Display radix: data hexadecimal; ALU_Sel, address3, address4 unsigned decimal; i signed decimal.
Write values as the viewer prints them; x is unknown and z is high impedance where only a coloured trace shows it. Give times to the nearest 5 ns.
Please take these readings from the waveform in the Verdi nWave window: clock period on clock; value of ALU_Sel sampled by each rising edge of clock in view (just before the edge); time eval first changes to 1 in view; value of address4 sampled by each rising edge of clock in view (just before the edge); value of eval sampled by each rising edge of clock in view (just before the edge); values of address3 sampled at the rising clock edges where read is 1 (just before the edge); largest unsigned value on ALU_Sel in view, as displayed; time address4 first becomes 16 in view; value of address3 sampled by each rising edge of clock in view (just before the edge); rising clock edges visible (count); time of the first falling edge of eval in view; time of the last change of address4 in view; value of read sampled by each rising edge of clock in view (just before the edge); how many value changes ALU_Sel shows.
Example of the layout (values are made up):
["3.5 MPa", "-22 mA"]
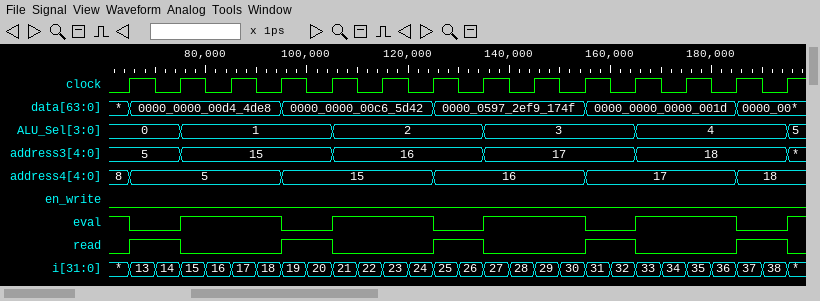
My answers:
["10 ns", "0, 0, 1, 1, 1, 2, 2, 2, 3, 3, 3, 4, 4, 4", "75 ns", "8, 5, 5, 5, 15, 15, 15, 16, 16, 16, 17, 17, 17, 18", "1 0 1 1 0 1 1 0 1 1 0 1 1 0", "5, 15, 16, 17, 18", "5", "125 ns", "5, 5, 15, 15, 15, 16, 16, 16, 17, 17, 17, 18, 18, 18", "14", "65 ns", "185 ns", "0 1 0 0 1 0 0 1 0 0 1 0 0 1", "5"]
